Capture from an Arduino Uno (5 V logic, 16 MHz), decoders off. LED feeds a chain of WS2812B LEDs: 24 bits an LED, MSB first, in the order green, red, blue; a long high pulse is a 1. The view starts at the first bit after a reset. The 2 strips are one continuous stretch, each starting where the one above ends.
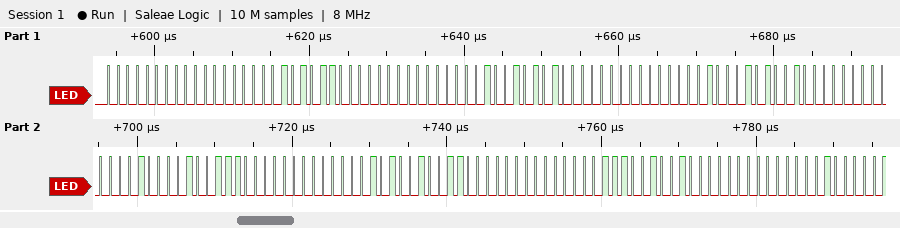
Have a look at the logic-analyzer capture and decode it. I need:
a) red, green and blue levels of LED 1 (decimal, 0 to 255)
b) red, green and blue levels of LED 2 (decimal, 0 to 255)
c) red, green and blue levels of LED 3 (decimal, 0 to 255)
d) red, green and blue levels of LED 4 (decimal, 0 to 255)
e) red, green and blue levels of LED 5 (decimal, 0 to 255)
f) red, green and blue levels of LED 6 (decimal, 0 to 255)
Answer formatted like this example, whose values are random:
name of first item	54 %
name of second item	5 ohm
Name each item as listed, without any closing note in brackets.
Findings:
red, green and blue levels of LED 1	0, 0, 43
red, green and blue levels of LED 2	1, 0, 42
red, green and blue levels of LED 3	2, 0, 41
red, green and blue levels of LED 4	4, 0, 39
red, green and blue levels of LED 5	5, 0, 38
red, green and blue levels of LED 6	7, 0, 36
